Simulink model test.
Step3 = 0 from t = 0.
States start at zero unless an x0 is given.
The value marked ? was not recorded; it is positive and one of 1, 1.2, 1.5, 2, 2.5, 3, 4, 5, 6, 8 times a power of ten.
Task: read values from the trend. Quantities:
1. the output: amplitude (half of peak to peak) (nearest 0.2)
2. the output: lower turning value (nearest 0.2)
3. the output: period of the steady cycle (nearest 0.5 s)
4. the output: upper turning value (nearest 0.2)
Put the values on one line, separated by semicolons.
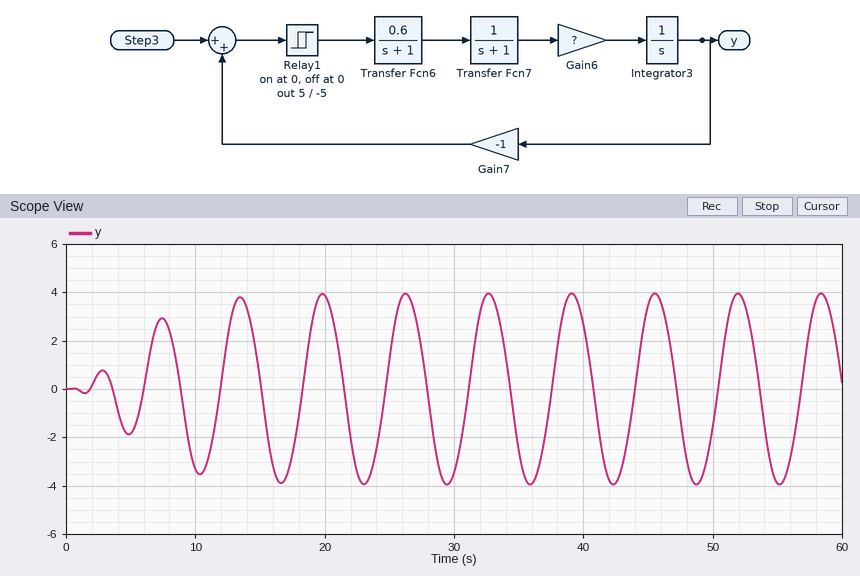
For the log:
4.0; -4.0; 6.5 s; 4.0
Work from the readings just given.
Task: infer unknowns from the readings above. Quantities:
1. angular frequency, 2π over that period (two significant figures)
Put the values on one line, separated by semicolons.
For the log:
0.97 rad/s
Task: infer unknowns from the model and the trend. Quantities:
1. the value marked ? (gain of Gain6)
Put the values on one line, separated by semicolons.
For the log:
2
